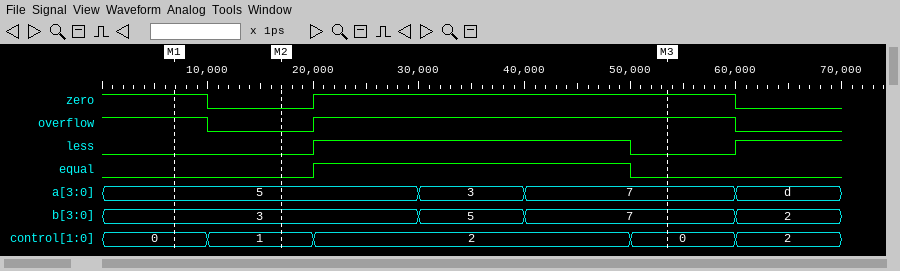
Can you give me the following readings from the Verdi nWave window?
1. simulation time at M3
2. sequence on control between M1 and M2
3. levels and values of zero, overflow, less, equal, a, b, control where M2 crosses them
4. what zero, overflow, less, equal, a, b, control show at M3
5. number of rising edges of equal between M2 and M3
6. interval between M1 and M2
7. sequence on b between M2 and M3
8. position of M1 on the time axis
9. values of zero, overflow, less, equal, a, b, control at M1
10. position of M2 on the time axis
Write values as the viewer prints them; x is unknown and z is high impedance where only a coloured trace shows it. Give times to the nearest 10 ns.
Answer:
50 ns
0, 1
zero=0, overflow=0, less=0, equal=0, a=5, b=3, control=1
zero=1, overflow=1, less=0, equal=0, a=7, b=7, control=0
1
10 ns
3, 5, 7
10 ns
zero=1, overflow=1, less=0, equal=0, a=5, b=3, control=0
20 ns
